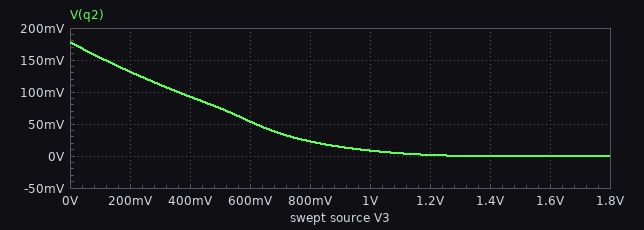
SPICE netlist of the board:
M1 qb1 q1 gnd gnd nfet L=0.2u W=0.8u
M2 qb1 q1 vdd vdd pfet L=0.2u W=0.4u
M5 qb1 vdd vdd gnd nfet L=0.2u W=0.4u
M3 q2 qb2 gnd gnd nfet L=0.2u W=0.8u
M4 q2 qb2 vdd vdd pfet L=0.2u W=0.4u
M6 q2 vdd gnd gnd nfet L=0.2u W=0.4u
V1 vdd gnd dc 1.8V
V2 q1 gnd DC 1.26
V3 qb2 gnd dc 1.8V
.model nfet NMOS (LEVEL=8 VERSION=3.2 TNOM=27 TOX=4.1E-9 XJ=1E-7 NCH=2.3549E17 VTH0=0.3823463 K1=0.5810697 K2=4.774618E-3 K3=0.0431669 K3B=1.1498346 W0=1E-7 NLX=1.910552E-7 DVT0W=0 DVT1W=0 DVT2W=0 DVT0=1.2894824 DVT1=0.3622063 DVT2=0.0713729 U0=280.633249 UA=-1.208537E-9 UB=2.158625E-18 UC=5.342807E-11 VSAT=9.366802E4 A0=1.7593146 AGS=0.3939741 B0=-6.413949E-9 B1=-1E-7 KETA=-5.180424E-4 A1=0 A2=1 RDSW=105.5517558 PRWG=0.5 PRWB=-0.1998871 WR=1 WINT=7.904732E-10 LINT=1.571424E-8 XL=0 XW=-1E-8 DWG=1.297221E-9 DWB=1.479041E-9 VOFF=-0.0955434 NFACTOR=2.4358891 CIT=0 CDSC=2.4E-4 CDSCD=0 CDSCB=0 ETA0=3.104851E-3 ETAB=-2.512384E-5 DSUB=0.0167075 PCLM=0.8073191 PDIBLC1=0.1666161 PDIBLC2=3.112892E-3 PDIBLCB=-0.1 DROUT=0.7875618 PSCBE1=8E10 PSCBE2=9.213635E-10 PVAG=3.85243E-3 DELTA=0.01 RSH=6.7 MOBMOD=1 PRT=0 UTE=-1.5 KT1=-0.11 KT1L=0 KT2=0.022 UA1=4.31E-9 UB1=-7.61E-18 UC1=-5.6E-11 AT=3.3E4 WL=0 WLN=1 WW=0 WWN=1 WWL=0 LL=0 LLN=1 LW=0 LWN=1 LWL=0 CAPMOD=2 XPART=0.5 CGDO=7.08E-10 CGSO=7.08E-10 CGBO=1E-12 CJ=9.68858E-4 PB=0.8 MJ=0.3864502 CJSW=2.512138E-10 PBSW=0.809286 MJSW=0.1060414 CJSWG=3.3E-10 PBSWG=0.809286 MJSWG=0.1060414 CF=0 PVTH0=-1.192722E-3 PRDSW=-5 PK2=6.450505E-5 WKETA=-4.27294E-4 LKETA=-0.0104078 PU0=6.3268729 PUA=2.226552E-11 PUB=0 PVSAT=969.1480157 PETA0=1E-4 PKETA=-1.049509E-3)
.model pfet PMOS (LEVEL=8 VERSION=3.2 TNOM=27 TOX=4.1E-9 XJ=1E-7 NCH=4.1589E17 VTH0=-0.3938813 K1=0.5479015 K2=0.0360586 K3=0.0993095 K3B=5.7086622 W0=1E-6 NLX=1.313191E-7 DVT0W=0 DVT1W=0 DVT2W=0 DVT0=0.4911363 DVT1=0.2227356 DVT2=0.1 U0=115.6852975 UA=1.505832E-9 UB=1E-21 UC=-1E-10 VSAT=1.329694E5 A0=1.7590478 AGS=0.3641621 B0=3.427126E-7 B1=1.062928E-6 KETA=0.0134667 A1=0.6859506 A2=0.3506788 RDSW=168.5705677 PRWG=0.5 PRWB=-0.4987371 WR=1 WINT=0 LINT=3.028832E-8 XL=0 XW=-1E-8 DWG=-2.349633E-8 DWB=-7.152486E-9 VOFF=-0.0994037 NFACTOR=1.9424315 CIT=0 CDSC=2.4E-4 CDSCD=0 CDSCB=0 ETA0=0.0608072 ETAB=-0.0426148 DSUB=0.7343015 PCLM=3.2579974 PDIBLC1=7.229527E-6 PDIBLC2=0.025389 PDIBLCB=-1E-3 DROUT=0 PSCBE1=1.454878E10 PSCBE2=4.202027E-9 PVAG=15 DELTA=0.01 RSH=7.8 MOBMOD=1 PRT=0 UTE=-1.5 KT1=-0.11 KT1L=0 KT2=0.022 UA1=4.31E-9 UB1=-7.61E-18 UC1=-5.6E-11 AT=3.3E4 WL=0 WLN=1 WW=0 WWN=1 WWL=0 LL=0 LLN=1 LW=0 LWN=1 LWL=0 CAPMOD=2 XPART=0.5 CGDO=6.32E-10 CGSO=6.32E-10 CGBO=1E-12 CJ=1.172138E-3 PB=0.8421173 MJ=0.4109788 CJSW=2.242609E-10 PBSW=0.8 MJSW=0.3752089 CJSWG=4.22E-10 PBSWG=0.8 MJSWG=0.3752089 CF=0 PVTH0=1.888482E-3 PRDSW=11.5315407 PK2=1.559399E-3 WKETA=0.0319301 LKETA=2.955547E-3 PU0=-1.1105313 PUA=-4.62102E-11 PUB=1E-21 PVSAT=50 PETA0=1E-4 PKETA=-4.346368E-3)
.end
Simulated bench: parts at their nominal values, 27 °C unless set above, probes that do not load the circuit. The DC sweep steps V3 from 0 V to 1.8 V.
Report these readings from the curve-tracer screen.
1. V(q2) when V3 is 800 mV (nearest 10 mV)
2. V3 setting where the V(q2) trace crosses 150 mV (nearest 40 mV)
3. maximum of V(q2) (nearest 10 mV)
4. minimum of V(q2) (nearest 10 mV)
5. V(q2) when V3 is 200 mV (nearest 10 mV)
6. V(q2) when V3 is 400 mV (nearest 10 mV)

20 mV
120 mV
180 mV
0 V
130 mV
90 mV
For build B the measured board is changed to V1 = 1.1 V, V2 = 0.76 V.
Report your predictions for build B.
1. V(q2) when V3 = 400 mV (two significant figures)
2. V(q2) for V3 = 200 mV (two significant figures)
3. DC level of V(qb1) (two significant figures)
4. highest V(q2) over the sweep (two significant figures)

13 mV
41 mV
200 mV
83 mV
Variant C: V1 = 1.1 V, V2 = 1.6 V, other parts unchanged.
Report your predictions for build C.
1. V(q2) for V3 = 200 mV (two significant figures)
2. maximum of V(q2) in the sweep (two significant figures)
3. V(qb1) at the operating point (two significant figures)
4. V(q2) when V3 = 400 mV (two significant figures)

41 mV
83 mV
61 mV
13 mV
